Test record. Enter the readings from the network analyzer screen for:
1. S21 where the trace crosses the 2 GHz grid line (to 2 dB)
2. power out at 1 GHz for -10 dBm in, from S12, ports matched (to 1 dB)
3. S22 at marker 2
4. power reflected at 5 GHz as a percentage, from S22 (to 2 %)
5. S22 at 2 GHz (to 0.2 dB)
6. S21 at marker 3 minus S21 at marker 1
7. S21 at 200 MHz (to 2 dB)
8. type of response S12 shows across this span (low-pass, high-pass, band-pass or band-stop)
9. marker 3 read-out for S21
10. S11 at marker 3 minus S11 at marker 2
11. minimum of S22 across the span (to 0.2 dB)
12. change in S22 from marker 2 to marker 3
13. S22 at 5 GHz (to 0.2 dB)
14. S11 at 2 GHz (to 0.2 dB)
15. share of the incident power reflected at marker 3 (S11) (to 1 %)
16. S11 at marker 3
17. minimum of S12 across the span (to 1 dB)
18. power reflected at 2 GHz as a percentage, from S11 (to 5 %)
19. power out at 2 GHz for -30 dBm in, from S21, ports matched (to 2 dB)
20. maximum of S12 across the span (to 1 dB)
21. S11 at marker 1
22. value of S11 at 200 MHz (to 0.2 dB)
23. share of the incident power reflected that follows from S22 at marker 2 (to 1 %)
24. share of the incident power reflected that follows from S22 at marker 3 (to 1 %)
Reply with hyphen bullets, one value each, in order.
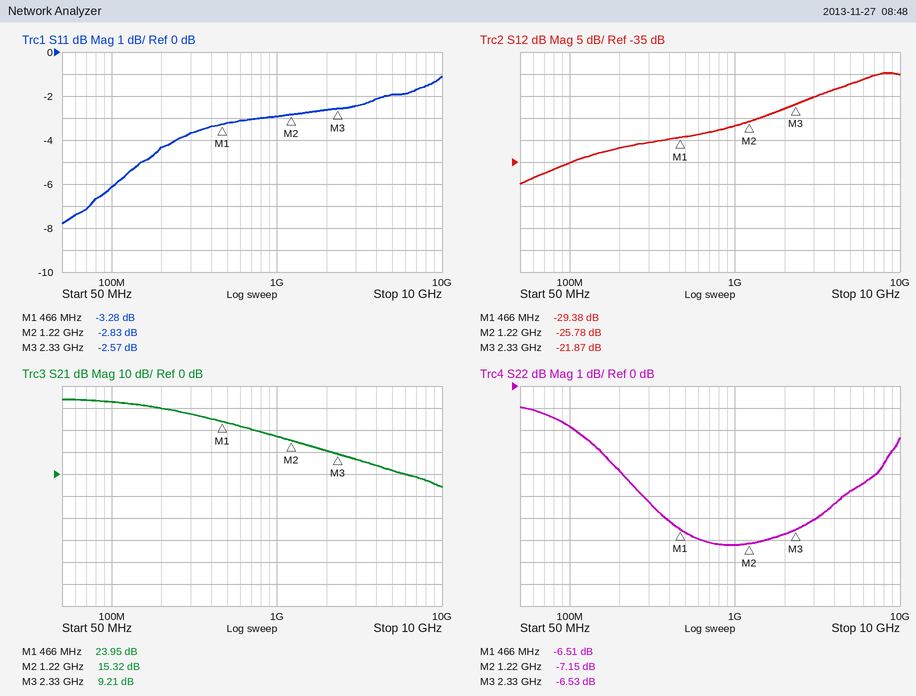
- 10 dB
- -37 dBm
- -7.15 dB
- 34 %
- -6.8 dB
- -14.74 dB
- 30 dB
- high-pass
- 9.21 dB
- 0.26 dB
- -7.2 dB
- 0.62 dB
- -4.8 dB
- -2.6 dB
- 55 %
- -2.57 dB
- -40 dB
- 55 %
- -20 dBm
- -15 dB
- -3.28 dB
- -4.4 dB
- 19 %
- 22 %
